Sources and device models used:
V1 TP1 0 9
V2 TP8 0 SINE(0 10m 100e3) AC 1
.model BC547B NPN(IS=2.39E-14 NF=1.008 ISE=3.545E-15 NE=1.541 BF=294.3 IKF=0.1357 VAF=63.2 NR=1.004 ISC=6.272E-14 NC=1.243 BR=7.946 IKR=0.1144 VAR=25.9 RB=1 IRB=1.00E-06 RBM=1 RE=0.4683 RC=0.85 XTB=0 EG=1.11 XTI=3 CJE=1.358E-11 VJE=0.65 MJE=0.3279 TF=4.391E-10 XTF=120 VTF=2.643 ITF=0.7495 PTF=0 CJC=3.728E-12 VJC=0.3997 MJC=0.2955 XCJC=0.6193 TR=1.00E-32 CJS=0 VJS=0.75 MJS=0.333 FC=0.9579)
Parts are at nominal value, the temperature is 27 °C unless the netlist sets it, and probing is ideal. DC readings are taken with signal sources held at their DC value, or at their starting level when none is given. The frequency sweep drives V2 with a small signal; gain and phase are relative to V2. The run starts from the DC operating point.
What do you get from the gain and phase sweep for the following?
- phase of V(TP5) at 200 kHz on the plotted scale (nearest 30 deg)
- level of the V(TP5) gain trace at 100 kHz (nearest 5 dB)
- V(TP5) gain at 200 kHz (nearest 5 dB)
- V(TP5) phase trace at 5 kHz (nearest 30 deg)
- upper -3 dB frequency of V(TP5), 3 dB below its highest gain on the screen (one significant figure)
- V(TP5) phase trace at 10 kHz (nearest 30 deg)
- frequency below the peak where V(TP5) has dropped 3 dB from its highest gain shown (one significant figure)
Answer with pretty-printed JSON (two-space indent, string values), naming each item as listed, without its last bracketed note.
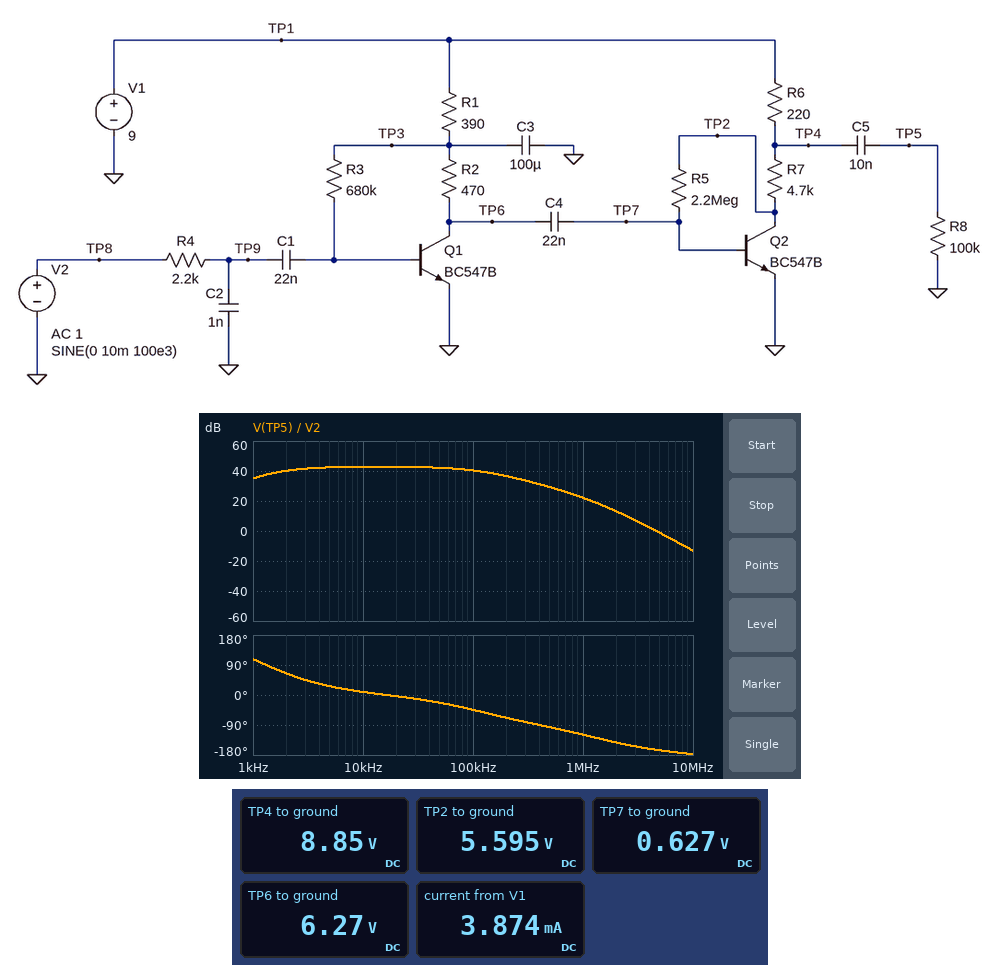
{
  "phase of V(TP5) at 200 kHz on the plotted scale": "-60 deg",
  "level of the V(TP5) gain trace at 100 kHz": "40 dB",
  "V(TP5) gain at 200 kHz": "35 dB",
  "V(TP5) phase trace at 5 kHz": "30 deg",
  "upper -3 dB frequency of V(TP5), 3 dB below its highest gain on the screen": "100 kHz",
  "V(TP5) phase trace at 10 kHz": "0 deg",
  "frequency below the peak where V(TP5) has dropped 3 dB from its highest gain shown": "2 kHz"
}
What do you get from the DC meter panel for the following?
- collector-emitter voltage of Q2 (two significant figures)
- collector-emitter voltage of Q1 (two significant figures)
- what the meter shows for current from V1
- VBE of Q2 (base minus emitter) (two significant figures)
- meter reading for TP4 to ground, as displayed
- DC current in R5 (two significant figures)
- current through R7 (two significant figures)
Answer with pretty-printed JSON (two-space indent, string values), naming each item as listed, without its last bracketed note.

{
  "collector-emitter voltage of Q2": "5.6 V",
  "collector-emitter voltage of Q1": "6.3 V",
  "what the meter shows for current from V1": "3.874 mA",
  "VBE of Q2 (base minus emitter)": "630 mV",
  "meter reading for TP4 to ground, as displayed": "8.85 V",
  "DC current in R5": "2.3 µA",
  "current through R7": "690 µA"
}
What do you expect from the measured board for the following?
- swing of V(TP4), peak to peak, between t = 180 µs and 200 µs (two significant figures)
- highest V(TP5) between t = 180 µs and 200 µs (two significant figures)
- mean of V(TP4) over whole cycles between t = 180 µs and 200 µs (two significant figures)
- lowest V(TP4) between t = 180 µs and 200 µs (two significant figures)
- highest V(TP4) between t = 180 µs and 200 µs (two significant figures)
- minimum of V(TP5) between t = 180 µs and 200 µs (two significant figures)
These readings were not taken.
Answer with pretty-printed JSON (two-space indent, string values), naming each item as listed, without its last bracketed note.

{
  "swing of V(TP4), peak to peak, between t = 180 µs and 200 µs": "400 mV",
  "highest V(TP5) between t = 180 µs and 200 µs": "150 mV",
  "mean of V(TP4) over whole cycles between t = 180 µs and 200 µs": "8.9 V",
  "lowest V(TP4) between t = 180 µs and 200 µs": "8.6 V",
  "highest V(TP4) between t = 180 µs and 200 µs": "9.0 V",
  "minimum of V(TP5) between t = 180 µs and 200 µs": "-250 mV"
}
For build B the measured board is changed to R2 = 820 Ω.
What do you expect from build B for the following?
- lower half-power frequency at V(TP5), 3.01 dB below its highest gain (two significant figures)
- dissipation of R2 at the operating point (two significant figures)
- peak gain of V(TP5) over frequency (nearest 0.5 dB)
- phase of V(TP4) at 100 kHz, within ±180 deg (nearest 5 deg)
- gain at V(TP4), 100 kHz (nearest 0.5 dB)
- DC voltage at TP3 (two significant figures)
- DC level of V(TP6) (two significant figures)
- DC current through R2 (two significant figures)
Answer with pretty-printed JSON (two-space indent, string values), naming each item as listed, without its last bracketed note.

{
  "lower half-power frequency at V(TP5), 3.01 dB below its highest gain": "1.8 kHz",
  "dissipation of R2 at the operating point": "8.0 mW",
  "peak gain of V(TP5) over frequency": "47.0 dB",
  "phase of V(TP4) at 100 kHz, within ±180 deg": "-50 deg",
  "gain at V(TP4), 100 kHz": "44.5 dB",
  "DC voltage at TP3": "7.8 V",
  "DC level of V(TP6)": "5.2 V",
  "DC current through R2": "3.1 mA"
}
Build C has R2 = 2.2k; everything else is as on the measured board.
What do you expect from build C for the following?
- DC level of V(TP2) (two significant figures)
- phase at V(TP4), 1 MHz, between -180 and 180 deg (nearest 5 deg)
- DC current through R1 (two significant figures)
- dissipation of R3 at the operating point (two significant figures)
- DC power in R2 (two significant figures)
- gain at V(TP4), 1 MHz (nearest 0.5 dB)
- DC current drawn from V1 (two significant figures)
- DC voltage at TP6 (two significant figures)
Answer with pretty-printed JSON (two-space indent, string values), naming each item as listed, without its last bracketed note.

{
  "DC level of V(TP2)": "5.6 V",
  "phase at V(TP4), 1 MHz, between -180 and 180 deg": "-145 deg",
  "DC current through R1": "3.0 mA",
  "dissipation of R3 at the operating point": "76 µW",
  "DC power in R2": "19 mW",
  "gain at V(TP4), 1 MHz": "25.5 dB",
  "DC current drawn from V1": "3.7 mA",
  "DC voltage at TP6": "1.3 V"
}
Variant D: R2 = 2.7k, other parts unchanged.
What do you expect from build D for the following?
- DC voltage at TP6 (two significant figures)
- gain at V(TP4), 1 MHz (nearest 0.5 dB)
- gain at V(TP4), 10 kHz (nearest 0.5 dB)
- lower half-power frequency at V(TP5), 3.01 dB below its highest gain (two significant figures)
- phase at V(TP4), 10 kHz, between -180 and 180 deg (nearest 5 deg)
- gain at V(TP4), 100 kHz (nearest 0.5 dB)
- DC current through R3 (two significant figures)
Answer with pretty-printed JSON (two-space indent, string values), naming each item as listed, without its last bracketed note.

{
  "DC voltage at TP6": "200 mV",
  "gain at V(TP4), 1 MHz": "20.0 dB",
  "gain at V(TP4), 10 kHz": "42.5 dB",
  "lower half-power frequency at V(TP5), 3.01 dB below its highest gain": "2.8 kHz",
  "phase at V(TP4), 10 kHz, between -180 and 180 deg": "15 deg",
  "gain at V(TP4), 100 kHz": "39.0 dB",
  "DC current through R3": "11 µA"
}
